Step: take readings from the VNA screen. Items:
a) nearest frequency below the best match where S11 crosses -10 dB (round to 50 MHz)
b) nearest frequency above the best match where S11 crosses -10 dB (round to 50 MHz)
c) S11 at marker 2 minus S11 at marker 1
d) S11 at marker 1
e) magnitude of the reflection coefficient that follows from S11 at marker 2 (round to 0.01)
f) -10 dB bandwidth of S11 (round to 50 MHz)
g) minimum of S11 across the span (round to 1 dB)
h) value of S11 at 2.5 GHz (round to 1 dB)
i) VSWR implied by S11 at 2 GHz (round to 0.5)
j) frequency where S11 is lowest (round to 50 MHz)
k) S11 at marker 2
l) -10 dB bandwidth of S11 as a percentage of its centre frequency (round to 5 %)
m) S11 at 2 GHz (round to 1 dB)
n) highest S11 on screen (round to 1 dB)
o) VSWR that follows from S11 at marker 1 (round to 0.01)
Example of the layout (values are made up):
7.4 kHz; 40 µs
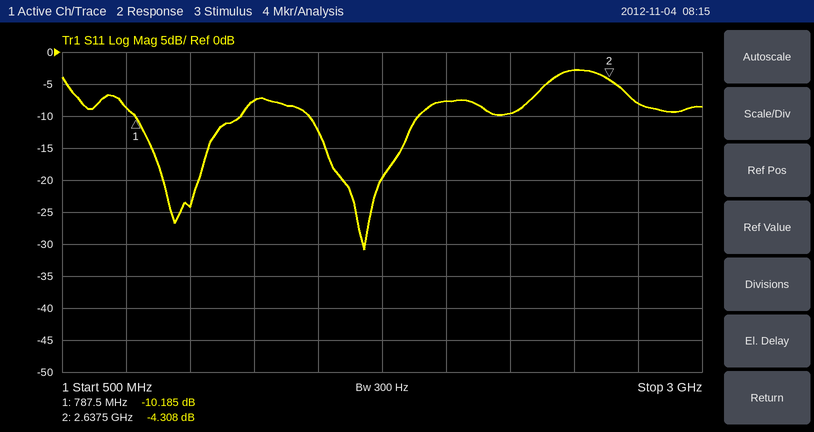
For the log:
1.45 GHz; 1.90 GHz; 5.877 dB; -10.185 dB; 0.61; 450 MHz; -31 dB; -3 dB; 2.5; 1.70 GHz; -4.308 dB; 25 %; -8 dB; -3 dB; 1.90
